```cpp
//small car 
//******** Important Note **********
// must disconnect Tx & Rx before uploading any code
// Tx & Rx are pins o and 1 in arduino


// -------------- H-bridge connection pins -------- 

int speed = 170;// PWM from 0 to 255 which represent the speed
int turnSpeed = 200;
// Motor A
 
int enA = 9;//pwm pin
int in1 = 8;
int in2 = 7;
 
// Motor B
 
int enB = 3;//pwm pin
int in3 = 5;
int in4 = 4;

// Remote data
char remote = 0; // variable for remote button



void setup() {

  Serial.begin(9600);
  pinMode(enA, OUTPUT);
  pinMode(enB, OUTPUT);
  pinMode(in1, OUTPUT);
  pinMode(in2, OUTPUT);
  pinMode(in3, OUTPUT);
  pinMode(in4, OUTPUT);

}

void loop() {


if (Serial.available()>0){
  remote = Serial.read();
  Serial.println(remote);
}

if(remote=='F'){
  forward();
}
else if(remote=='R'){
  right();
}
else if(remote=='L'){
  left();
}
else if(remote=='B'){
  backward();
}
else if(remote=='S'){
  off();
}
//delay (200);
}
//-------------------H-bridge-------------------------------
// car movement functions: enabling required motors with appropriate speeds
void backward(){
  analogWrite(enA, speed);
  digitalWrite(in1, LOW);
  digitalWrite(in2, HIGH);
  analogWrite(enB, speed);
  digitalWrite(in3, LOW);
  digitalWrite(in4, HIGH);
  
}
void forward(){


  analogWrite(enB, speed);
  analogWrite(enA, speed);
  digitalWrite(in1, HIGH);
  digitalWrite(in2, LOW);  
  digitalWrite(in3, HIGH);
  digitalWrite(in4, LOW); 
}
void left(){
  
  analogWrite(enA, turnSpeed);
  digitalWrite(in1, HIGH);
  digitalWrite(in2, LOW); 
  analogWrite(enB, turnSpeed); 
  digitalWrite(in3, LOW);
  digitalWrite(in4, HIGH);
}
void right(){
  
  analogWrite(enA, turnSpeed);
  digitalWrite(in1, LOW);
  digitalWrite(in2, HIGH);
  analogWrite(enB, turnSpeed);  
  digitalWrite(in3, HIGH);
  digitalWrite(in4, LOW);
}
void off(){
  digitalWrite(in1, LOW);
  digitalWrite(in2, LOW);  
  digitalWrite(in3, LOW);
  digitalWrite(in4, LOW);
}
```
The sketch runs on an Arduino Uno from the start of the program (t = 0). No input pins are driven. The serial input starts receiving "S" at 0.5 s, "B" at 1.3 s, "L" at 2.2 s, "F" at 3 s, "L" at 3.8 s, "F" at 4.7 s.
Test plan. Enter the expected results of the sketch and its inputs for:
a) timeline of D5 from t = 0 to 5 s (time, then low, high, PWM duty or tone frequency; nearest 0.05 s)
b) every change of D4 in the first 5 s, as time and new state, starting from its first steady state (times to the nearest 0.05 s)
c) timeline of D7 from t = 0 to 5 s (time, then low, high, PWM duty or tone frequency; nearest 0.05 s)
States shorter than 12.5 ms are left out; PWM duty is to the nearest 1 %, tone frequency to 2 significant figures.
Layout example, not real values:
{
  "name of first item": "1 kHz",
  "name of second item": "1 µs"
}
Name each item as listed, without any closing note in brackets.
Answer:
{
  "timeline of D5 from t = 0 to 5 s": "0 s low; 3 s high; 3.8 s low; 4.7 s high",
  "every change of D4 in the first 5 s, as time and new state, starting from its first steady state": "0 s low; 1.3 s high; 3 s low; 3.8 s high; 4.7 s low",
  "timeline of D7 from t = 0 to 5 s": "0 s low; 1.3 s high; 2.2 s low"
}
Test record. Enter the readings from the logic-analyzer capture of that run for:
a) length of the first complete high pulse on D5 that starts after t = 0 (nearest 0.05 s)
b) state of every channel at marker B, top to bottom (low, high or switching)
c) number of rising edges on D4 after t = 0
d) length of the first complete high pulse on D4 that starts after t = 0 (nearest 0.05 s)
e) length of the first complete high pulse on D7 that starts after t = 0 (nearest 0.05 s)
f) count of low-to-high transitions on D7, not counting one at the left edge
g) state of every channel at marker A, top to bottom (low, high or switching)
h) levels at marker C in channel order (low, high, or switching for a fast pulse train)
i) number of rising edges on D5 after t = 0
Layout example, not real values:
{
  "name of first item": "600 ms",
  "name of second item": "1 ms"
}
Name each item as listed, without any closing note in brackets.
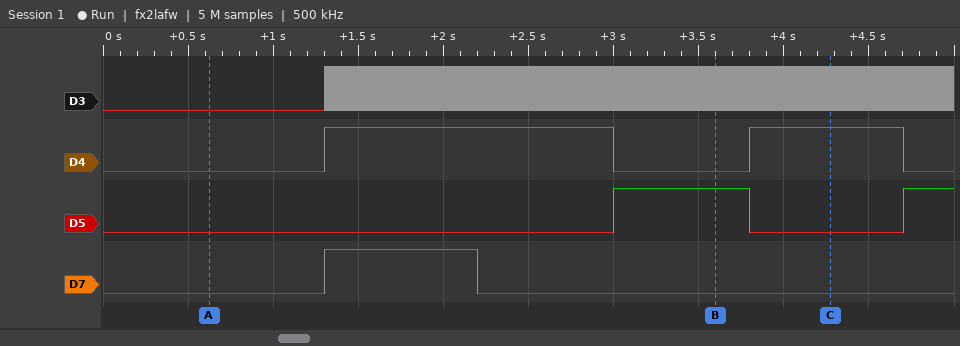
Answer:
{
  "length of the first complete high pulse on D5 that starts after t = 0": "0.80 s",
  "state of every channel at marker B, top to bottom": "D3 switching, D4 low, D5 high, D7 low",
  "number of rising edges on D4 after t = 0": "2",
  "length of the first complete high pulse on D4 that starts after t = 0": "1.70 s",
  "length of the first complete high pulse on D7 that starts after t = 0": "0.90 s",
  "count of low-to-high transitions on D7, not counting one at the left edge": "1",
  "state of every channel at marker A, top to bottom": "D3 low, D4 low, D5 low, D7 low",
  "levels at marker C in channel order": "D3 switching, D4 high, D5 low, D7 low",
  "number of rising edges on D5 after t = 0": "2"
}
